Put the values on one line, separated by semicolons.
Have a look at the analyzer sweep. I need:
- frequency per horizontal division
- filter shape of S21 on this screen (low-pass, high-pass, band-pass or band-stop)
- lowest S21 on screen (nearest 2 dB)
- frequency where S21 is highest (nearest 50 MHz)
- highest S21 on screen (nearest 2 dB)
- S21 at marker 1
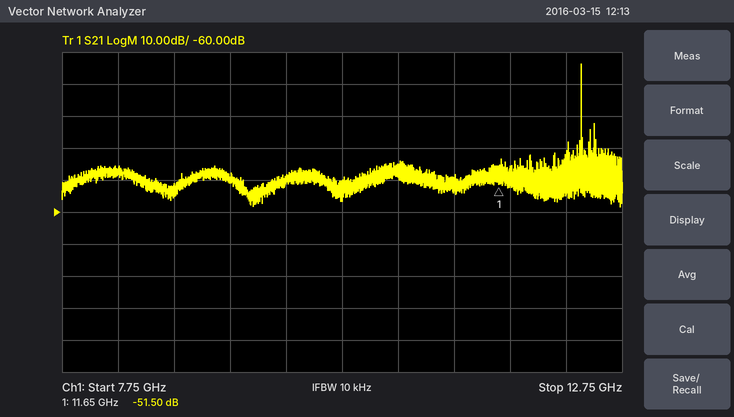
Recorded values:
500 MHz; band-pass; -58 dB; 12.40 GHz; -14 dB; -51.50 dB
